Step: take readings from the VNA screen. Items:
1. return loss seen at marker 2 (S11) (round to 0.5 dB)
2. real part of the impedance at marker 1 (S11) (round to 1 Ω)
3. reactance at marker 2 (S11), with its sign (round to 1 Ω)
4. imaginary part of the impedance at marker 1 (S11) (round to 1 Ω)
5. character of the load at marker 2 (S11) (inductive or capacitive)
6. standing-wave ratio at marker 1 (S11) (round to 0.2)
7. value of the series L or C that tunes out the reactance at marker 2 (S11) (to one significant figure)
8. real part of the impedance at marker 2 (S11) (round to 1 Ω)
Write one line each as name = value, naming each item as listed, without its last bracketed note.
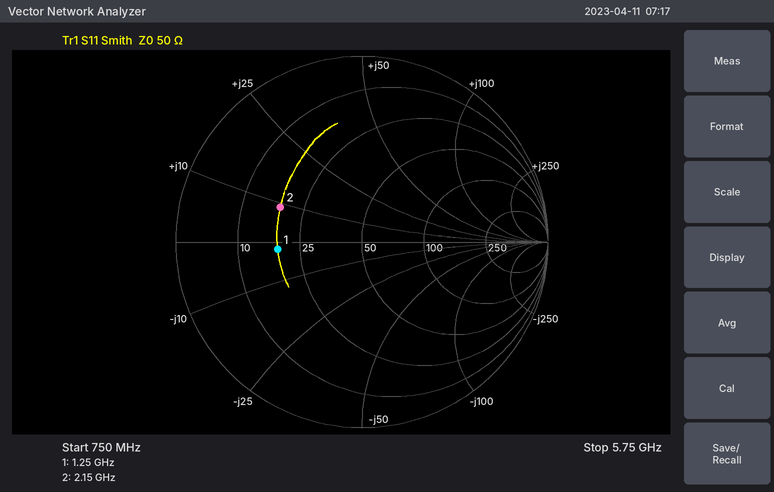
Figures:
return loss seen at marker 2 (S11) = 6.5 dB
real part of the impedance at marker 1 (S11) = 19 Ω
reactance at marker 2 (S11), with its sign = +9 Ω
imaginary part of the impedance at marker 1 (S11) = -2 Ω
character of the load at marker 2 (S11) = inductive
standing-wave ratio at marker 1 (S11) = 2.6
value of the series L or C that tunes out the reactance at marker 2 (S11) = 8 pF
real part of the impedance at marker 2 (S11) = 18 Ω
